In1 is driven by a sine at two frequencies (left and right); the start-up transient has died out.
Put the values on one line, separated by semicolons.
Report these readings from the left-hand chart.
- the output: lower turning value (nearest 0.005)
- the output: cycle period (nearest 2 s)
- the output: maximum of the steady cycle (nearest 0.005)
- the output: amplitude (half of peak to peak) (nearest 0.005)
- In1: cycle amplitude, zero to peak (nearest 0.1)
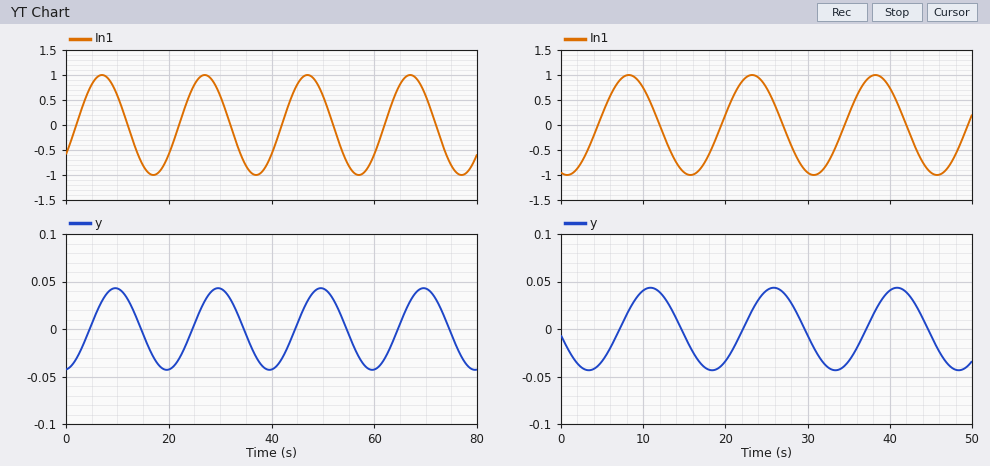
-0.045; 20 s; 0.045; 0.045; 1.0
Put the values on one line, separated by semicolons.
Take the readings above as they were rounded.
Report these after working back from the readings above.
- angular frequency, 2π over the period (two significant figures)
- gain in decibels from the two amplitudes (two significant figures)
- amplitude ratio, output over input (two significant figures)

0.31 rad/s; -27 dB; 0.045
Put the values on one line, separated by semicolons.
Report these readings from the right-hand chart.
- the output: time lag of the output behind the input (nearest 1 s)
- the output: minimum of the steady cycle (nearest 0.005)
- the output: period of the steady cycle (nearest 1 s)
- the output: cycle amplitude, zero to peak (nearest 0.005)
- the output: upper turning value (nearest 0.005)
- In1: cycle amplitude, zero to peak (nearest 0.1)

3 s; -0.045; 15 s; 0.045; 0.045; 1.0
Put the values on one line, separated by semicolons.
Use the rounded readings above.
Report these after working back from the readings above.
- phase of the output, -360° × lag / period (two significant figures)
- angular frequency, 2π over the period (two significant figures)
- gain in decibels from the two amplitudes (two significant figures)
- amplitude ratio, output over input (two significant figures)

-72°; 0.42 rad/s; -27 dB; 0.045
